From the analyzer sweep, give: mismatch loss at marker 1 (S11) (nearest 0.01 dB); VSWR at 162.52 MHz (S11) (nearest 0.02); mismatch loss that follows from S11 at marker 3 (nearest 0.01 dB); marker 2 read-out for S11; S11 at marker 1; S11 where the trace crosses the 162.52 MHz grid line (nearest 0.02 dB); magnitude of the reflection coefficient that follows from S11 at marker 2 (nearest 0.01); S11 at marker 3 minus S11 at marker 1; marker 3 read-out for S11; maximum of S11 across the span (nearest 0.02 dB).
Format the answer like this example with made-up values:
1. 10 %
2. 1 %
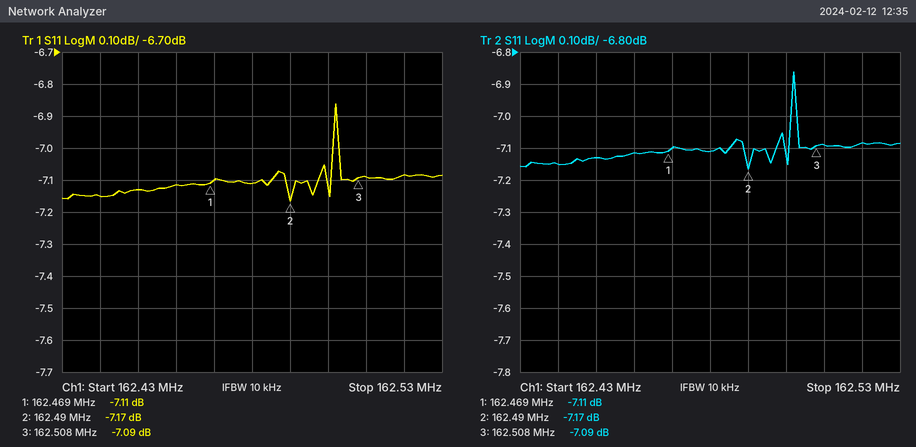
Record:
1. 0.94 dB
2. 2.58
3. 0.94 dB
4. -7.17 dB
5. -7.11 dB
6. -7.08 dB
7. 0.44
8. 0.02 dB
9. -7.09 dB
10. -6.86 dB
